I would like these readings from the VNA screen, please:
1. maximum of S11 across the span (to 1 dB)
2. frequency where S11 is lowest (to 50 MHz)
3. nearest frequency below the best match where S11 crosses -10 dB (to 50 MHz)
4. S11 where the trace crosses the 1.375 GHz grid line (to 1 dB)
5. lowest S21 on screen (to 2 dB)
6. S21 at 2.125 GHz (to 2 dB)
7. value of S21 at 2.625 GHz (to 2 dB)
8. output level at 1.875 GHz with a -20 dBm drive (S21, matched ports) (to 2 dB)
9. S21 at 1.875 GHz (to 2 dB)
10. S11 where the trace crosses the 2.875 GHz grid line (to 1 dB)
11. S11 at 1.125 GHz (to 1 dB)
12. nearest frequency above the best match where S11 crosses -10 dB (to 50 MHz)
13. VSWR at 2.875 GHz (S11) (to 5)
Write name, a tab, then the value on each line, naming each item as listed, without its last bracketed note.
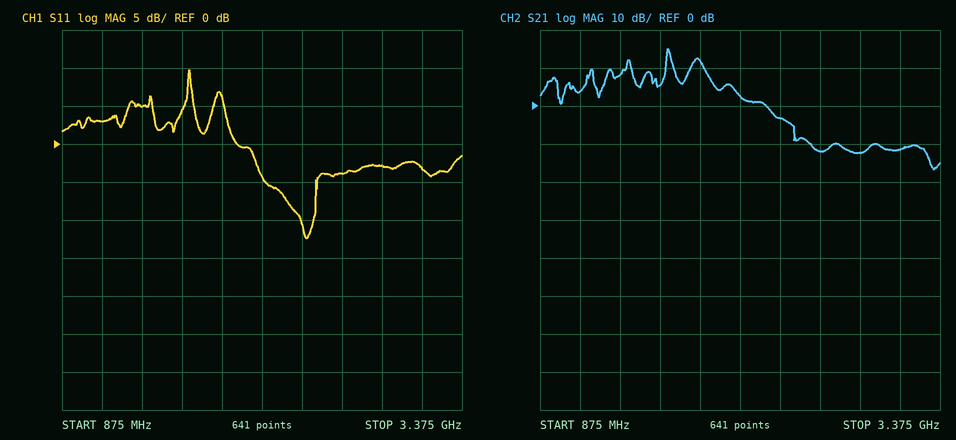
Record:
maximum of S11 across the span	10 dB
frequency where S11 is lowest	2.40 GHz
nearest frequency below the best match where S11 crosses -10 dB	2.35 GHz
S11 where the trace crosses the 1.375 GHz grid line	5 dB
lowest S21 on screen	-16 dB
S21 at 2.125 GHz	2 dB
value of S21 at 2.625 GHz	-12 dB
output level at 1.875 GHz with a -20 dBm drive (S21, matched ports)	-8 dBm
S21 at 1.875 GHz	12 dB
S11 where the trace crosses the 2.875 GHz grid line	-3 dB
S11 at 1.125 GHz	3 dB
nearest frequency above the best match where S11 crosses -10 dB	2.45 GHz
VSWR at 2.875 GHz (S11)	5
